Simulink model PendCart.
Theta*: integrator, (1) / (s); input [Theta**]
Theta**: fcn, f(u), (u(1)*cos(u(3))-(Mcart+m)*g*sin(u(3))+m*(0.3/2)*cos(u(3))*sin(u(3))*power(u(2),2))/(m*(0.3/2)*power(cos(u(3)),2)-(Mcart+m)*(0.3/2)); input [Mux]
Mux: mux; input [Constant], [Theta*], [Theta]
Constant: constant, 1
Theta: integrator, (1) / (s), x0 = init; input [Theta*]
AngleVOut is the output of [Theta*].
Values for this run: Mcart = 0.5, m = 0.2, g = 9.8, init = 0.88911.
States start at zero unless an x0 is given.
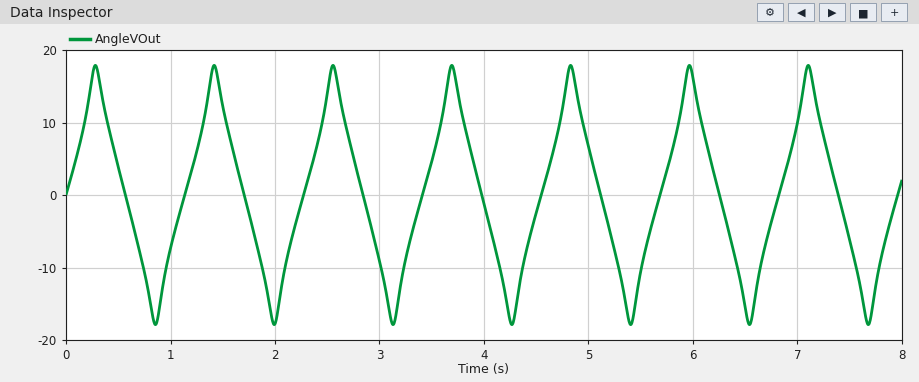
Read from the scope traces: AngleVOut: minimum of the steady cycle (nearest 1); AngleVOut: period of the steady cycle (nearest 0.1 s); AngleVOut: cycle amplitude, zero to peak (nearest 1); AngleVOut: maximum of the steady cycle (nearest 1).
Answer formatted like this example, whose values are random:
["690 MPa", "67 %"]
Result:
["-18", "1.1 s", "18", "18"]
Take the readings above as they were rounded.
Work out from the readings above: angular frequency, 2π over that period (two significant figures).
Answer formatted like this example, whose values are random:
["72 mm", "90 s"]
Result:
["5.7 rad/s"]
